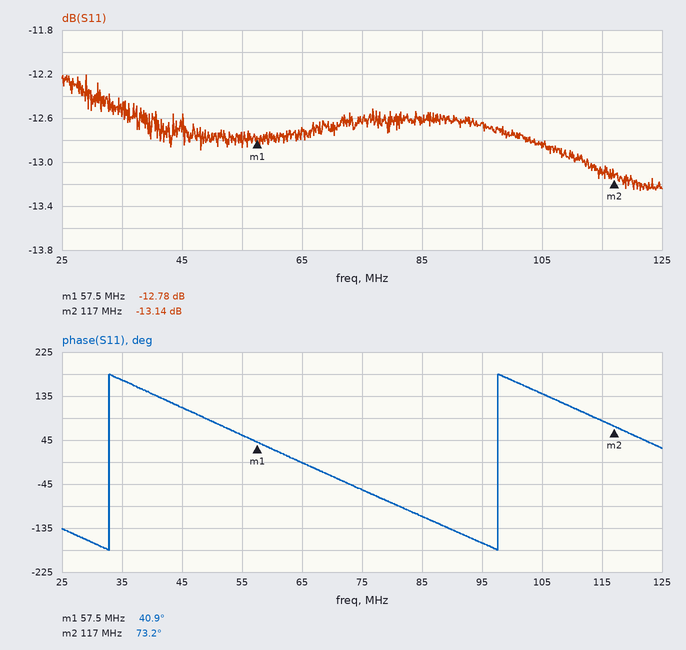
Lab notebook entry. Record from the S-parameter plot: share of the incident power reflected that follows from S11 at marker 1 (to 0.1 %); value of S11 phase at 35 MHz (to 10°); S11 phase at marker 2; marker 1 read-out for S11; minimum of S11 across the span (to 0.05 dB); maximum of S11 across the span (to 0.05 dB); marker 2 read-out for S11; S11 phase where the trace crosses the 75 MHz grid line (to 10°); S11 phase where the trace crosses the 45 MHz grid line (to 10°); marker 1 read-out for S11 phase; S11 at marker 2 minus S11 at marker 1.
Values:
5.3 %
170°
73.2°
-12.78 dB
-13.25 dB
-12.20 dB
-13.14 dB
-60°
110°
40.9°
-0.36 dB
